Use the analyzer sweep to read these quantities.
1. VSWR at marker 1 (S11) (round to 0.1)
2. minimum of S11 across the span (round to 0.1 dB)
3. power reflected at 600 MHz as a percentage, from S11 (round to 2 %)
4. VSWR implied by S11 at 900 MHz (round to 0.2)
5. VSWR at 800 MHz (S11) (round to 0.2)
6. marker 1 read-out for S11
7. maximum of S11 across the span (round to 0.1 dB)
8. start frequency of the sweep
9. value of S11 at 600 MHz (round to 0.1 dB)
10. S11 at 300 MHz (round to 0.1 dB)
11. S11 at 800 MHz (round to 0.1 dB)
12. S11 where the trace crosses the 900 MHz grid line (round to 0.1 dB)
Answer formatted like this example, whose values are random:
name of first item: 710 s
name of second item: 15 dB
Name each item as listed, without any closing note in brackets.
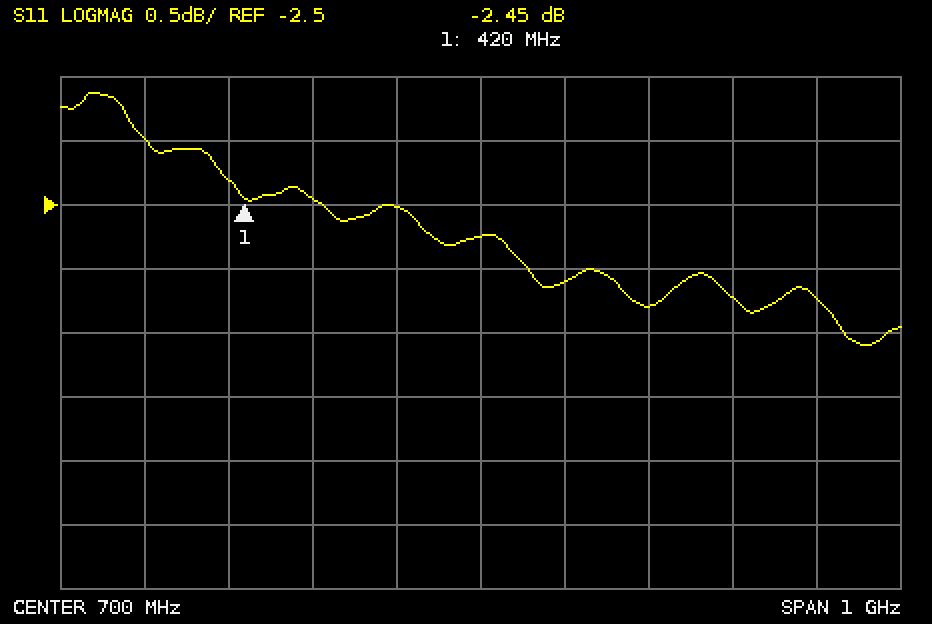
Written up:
VSWR at marker 1 (S11): 7.1
minimum of S11 across the span: -3.6 dB
power reflected at 600 MHz as a percentage, from S11: 56 %
VSWR implied by S11 at 900 MHz: 5.4
VSWR at 800 MHz (S11): 5.6
marker 1 read-out for S11: -2.45 dB
maximum of S11 across the span: -1.6 dB
start frequency of the sweep: 200 MHz
value of S11 at 600 MHz: -2.5 dB
S11 at 300 MHz: -2.0 dB
S11 at 800 MHz: -3.1 dB
S11 where the trace crosses the 900 MHz grid line: -3.3 dB
